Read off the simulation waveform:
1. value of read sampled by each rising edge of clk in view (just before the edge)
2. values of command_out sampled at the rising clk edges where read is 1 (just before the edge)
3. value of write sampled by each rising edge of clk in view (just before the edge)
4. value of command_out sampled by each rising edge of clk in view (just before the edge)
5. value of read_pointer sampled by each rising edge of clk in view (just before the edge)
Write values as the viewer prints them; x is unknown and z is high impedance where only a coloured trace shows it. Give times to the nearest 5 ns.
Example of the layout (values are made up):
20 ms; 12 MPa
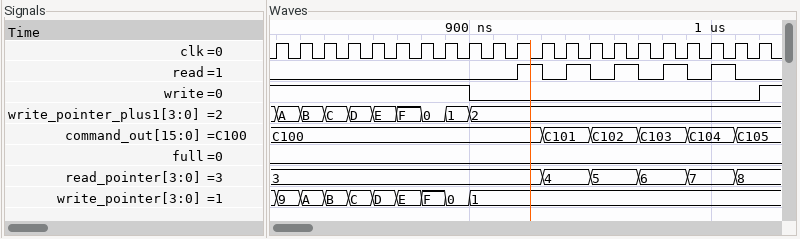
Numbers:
0 0 0 0 0 0 0 0 0 0 0 1 0 1 0 1 0 1 0 1 0; C100, C101, C102, C103, C104; 1 1 1 1 1 1 1 1 1 0 0 0 0 0 0 0 0 0 0 0 0; C100, C100, C100, C100, C100, C100, C100, C100, C100, C100, C100, C100, C101, C101, C102, C102, C103, C103, C104, C104, C105; 3, 3, 3, 3, 3, 3, 3, 3, 3, 3, 3, 3, 4, 4, 5, 5, 6, 6, 7, 7, 8
